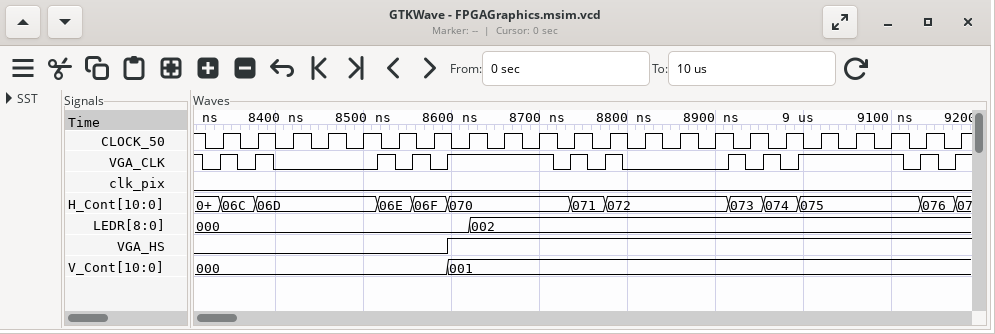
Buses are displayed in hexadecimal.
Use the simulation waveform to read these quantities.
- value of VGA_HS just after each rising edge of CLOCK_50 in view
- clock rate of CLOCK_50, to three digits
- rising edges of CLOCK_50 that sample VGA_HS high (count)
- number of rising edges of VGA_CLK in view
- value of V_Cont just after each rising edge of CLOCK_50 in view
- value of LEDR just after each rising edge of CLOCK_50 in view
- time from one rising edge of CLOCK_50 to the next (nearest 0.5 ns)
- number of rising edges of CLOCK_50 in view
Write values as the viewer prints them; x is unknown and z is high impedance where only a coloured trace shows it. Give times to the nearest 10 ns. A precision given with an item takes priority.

0 0 0 0 0 0 0 1 1 1 1 1 1 1 1 1 1 1 1 1 1 1
25.0 MHz
15
12
000, 000, 000, 000, 000, 000, 000, 001, 001, 001, 001, 001, 001, 001, 001, 001, 001, 001, 001, 001, 001, 001
000, 000, 000, 000, 000, 000, 000, 002, 002, 002, 002, 002, 002, 002, 002, 002, 002, 002, 002, 002, 002, 002
40 ns
22
